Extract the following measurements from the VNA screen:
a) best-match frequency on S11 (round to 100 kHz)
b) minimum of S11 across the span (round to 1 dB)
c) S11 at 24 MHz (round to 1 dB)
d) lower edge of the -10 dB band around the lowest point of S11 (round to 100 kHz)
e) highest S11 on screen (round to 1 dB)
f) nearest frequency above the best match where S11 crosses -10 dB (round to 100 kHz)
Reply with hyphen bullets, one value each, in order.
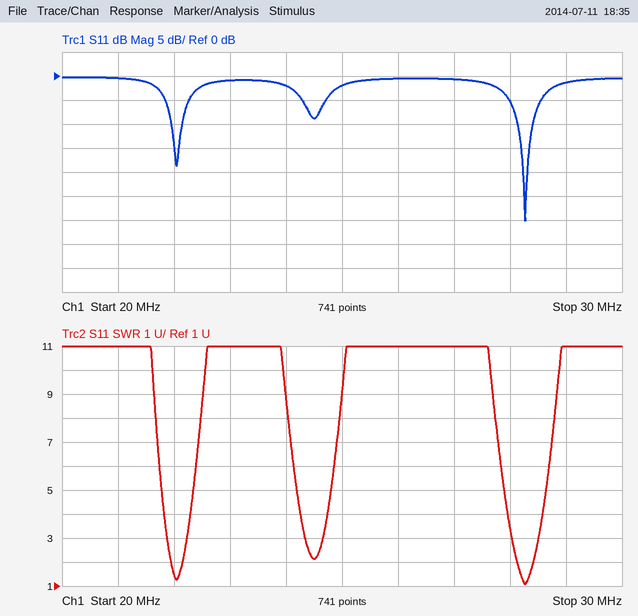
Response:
- 28.3 MHz
- -30 dB
- -2 dB
- 28.1 MHz
- 0 dB
- 28.4 MHz
